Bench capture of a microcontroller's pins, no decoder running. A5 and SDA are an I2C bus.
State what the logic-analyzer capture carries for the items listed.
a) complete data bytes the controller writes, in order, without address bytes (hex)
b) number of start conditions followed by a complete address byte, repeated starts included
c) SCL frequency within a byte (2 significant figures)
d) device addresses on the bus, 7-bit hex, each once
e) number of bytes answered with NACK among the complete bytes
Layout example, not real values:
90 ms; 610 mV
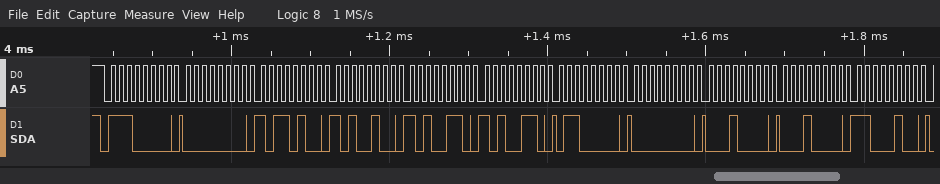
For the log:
00 B4 A4 A6 A6 60 00 10 10 C4; 1; 100 kHz; 0x70; 0
